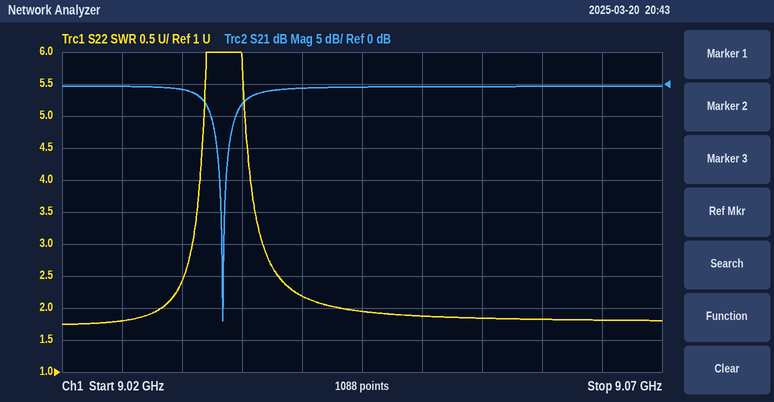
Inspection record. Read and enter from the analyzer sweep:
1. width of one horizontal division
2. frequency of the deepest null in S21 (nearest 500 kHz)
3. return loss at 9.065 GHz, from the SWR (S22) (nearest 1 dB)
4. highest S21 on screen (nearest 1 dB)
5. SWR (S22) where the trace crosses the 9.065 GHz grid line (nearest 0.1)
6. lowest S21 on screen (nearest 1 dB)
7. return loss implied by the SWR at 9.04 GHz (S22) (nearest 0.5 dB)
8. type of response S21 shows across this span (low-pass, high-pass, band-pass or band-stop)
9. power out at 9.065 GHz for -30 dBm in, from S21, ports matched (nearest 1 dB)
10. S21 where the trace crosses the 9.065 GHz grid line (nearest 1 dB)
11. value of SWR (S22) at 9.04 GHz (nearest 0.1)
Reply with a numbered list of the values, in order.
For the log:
1. 5 MHz
2. 9.0335 GHz
3. 11 dB
4. 0 dB
5. 1.8
6. -37 dB
7. 8.5 dB
8. band-stop
9. -30 dBm
10. 0 dB
11. 2.2
